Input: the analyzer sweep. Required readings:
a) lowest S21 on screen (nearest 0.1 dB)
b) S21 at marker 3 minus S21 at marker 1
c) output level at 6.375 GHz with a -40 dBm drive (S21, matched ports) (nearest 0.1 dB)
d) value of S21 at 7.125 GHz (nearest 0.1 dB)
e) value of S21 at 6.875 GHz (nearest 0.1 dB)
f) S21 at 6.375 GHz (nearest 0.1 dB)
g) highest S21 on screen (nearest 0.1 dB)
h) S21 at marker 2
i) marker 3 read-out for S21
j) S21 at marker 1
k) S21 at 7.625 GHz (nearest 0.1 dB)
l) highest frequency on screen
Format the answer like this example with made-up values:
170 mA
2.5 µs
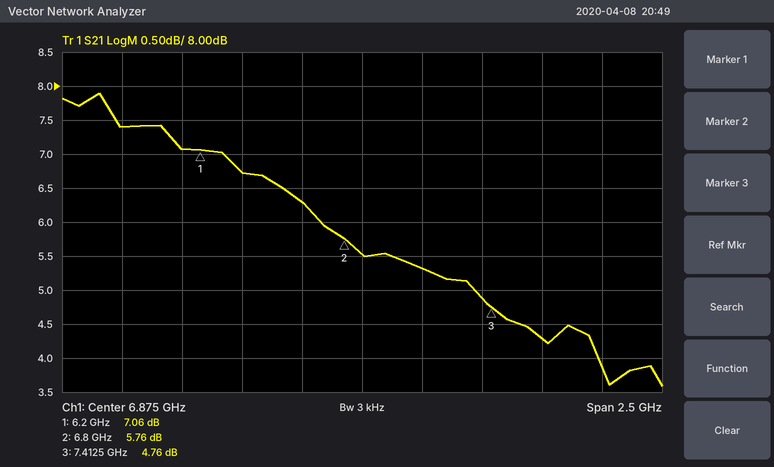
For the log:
3.6 dB
-2.30 dB
-33.3 dBm
5.3 dB
5.5 dB
6.7 dB
7.9 dB
5.76 dB
4.76 dB
7.06 dB
4.3 dB
8.125 GHz
